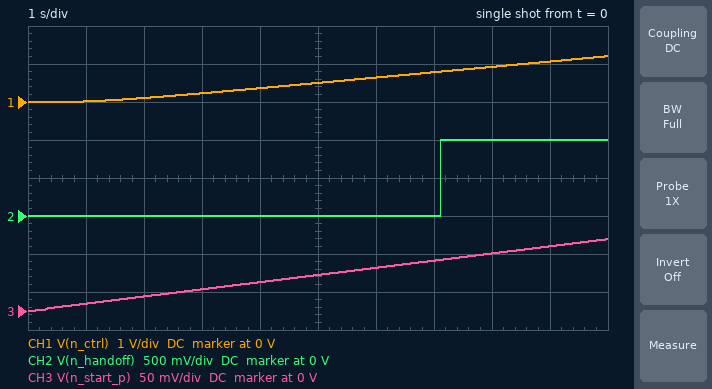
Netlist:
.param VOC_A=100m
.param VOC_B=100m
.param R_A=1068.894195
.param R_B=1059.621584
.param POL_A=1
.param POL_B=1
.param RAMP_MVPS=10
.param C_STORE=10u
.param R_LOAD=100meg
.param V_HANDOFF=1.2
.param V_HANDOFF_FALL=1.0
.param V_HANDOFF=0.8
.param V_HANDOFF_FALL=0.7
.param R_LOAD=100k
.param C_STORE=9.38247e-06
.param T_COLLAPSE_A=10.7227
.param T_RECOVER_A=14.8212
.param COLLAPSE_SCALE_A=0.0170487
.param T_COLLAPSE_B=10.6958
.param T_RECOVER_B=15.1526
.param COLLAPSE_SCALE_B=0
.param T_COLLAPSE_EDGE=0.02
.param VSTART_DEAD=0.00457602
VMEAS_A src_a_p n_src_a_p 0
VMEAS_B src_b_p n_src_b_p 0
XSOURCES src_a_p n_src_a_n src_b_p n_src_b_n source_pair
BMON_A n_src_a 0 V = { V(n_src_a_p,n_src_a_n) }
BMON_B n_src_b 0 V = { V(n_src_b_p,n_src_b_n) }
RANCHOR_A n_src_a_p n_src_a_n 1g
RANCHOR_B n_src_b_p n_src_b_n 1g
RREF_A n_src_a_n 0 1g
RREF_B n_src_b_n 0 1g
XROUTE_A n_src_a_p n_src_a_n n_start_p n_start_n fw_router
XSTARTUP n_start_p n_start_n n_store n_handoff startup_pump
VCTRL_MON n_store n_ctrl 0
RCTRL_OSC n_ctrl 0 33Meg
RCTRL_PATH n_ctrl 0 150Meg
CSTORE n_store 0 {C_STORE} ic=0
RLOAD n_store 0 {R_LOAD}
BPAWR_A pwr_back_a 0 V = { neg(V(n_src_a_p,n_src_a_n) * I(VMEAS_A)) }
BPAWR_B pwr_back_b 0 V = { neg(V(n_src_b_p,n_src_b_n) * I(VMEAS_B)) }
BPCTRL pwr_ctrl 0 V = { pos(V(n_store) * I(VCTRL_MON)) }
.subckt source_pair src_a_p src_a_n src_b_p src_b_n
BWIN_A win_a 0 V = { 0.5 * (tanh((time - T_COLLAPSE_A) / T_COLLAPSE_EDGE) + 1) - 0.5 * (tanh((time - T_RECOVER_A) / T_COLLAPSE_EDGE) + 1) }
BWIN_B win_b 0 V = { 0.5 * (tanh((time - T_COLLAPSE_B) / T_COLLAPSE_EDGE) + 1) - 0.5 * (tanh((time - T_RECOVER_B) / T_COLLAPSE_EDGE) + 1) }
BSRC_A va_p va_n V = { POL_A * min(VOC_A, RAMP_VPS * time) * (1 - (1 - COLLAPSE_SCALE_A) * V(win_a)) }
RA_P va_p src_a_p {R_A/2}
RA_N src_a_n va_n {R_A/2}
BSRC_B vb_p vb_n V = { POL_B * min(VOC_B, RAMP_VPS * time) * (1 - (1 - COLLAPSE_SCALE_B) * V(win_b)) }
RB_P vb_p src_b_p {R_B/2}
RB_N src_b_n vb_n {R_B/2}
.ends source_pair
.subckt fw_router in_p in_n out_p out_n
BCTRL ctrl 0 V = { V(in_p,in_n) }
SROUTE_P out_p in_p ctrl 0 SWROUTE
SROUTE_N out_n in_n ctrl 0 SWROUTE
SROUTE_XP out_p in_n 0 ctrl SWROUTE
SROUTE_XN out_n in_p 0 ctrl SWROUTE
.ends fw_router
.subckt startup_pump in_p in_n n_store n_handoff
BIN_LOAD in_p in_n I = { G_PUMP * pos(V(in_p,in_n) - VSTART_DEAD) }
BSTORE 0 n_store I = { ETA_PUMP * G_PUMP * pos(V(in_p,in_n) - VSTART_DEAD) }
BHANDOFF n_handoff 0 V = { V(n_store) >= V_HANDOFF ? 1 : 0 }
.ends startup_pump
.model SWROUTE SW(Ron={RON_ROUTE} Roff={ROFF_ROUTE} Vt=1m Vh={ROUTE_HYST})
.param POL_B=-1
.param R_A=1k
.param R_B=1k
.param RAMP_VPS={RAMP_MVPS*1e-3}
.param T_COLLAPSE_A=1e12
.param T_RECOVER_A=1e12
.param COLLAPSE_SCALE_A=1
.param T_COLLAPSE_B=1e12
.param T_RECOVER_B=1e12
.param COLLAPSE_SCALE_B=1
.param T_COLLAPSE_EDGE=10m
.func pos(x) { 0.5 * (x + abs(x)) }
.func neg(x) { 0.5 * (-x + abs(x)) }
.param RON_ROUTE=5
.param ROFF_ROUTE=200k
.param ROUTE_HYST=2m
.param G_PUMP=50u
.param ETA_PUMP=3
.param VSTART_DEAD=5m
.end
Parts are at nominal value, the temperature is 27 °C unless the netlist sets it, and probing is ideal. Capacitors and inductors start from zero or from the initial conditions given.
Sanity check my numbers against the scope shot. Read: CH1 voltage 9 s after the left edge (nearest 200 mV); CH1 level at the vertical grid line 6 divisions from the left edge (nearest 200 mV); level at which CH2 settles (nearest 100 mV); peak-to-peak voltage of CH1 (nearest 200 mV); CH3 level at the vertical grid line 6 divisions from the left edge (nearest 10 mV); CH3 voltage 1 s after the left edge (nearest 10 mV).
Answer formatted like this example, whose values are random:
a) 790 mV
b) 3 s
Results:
a) 1.0 V
b) 600 mV
c) 1.0 V
d) 1.2 V
e) 60 mV
f) 10 mV
